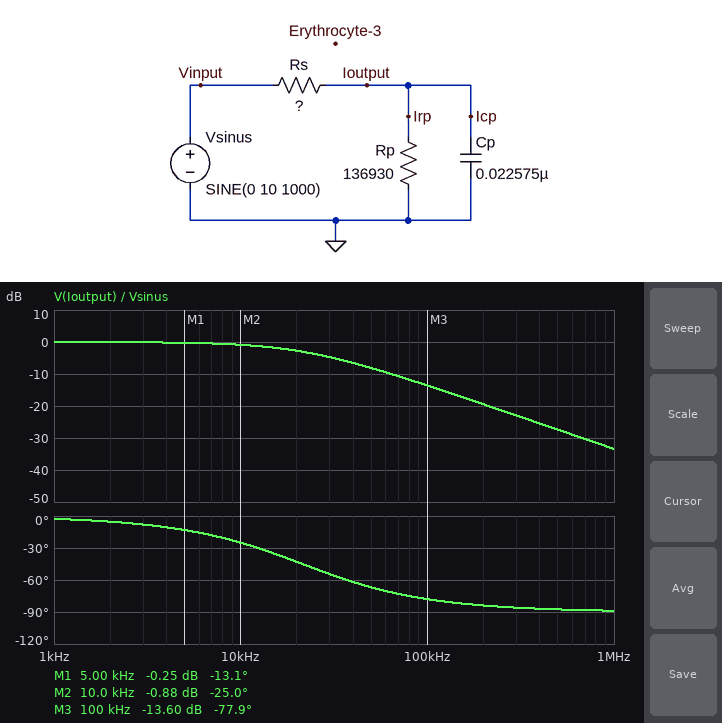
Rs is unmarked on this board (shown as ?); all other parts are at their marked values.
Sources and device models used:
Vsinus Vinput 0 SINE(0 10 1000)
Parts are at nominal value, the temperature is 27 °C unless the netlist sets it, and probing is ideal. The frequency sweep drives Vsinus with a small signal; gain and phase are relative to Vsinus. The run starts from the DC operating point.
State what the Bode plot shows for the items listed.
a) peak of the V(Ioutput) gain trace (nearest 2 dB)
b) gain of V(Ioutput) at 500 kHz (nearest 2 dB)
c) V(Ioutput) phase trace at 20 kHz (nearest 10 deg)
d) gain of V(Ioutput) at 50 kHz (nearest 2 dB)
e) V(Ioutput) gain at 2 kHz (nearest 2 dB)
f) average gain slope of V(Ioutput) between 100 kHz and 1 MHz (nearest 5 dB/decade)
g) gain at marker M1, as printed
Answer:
0 dB
-28 dB
-40 deg
-8 dB
0 dB
-20 dB/decade
-0.25 dB
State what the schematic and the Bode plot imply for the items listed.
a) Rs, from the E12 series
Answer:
330 Ω
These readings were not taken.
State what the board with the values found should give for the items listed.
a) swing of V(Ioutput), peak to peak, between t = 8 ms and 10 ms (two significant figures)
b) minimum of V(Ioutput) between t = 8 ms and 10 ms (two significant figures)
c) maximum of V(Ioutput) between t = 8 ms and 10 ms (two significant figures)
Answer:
20 V
-10 V
10 V
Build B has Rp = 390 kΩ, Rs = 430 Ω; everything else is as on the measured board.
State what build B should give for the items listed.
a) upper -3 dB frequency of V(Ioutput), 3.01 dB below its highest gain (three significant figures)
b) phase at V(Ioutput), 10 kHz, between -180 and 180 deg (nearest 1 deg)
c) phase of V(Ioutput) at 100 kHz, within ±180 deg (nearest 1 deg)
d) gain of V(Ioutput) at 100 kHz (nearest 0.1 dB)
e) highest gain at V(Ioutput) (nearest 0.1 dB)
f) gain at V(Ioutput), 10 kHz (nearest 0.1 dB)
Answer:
16.4 kHz
-31 deg
-81 deg
-15.8 dB
0 dB
-1.4 dB
